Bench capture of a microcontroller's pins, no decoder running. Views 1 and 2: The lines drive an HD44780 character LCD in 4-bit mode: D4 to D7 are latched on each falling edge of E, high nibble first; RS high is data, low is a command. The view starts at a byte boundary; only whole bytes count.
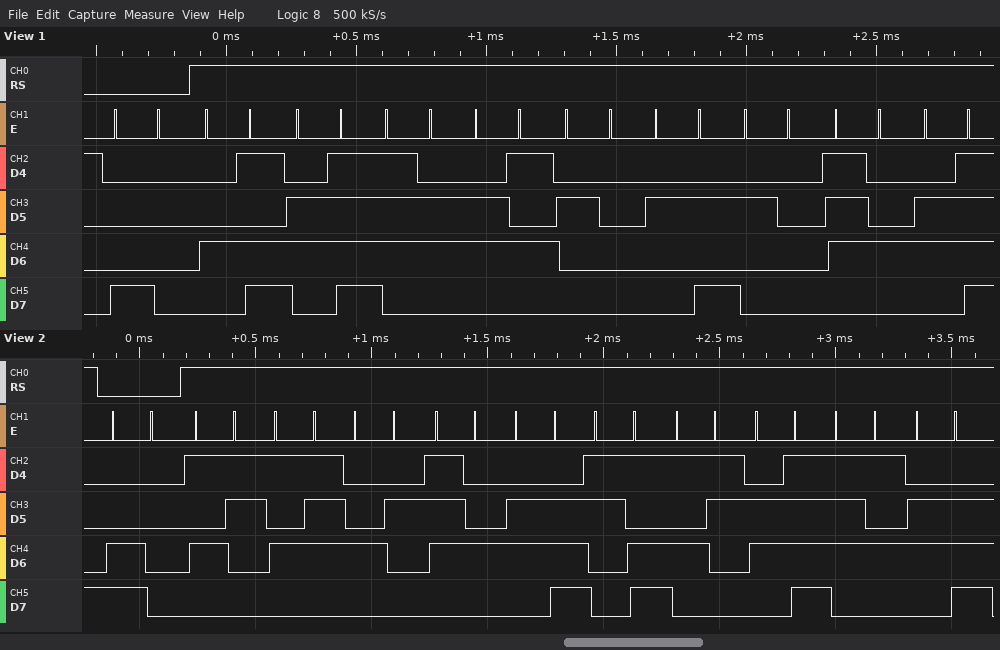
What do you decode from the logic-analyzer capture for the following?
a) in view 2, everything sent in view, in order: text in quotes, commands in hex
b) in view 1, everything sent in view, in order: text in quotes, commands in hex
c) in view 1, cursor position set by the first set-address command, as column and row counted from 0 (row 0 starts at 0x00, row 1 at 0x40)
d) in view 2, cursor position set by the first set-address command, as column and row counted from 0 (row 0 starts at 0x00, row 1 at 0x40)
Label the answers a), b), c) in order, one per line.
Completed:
a) 0xC0 "SWBtn=Soun"
b) 0x80 "Move * to"
c) column 0, row 0
d) column 0, row 1
